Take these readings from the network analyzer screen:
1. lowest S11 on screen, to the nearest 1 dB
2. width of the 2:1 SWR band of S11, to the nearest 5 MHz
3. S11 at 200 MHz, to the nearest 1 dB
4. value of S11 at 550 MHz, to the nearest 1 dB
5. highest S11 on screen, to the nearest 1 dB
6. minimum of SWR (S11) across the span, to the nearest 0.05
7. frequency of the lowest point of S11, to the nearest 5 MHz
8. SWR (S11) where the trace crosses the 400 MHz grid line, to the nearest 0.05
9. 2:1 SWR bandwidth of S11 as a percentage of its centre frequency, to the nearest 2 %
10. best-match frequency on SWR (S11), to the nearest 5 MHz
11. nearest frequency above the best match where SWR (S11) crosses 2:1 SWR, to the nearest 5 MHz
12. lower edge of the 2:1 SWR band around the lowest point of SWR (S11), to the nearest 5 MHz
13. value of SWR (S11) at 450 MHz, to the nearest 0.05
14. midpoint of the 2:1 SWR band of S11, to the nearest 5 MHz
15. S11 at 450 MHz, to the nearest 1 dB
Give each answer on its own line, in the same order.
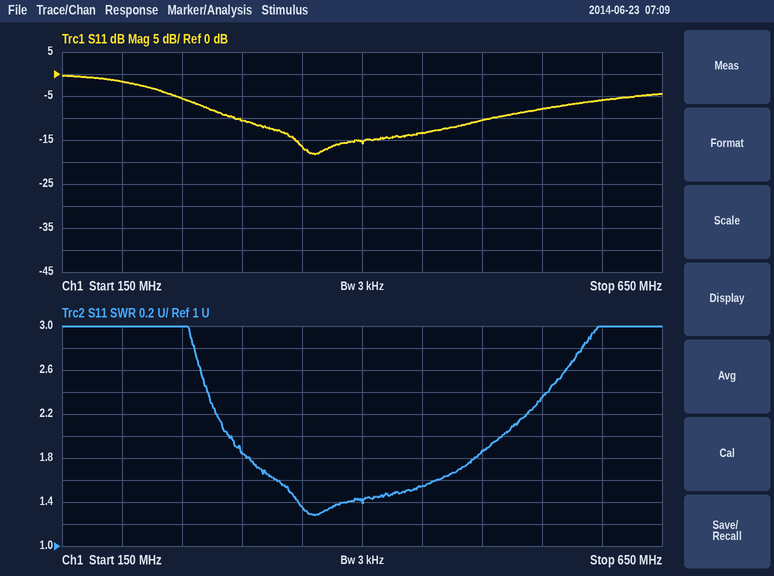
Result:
-18 dB
225 MHz
-2 dB
-8 dB
0 dB
1.30
360 MHz
1.40
56 %
360 MHz
515 MHz
290 MHz
1.55
405 MHz
-13 dB
